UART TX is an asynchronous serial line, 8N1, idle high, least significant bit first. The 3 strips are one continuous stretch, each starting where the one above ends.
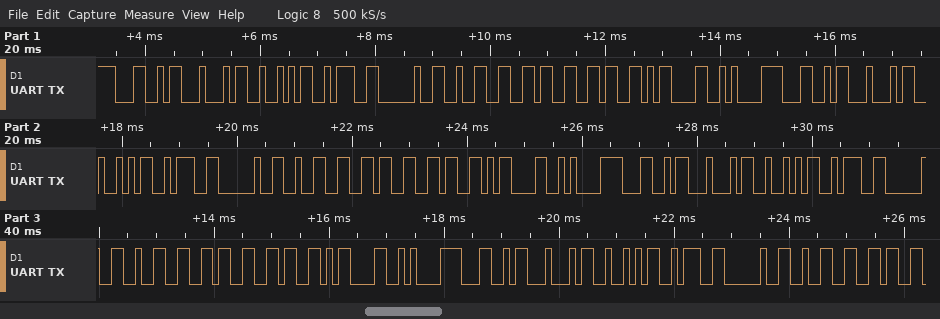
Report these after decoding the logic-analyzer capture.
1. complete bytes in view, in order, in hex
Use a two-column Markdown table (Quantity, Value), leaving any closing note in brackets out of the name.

| Quantity | Value |
|---|---|
| complete bytes in view, in order, in hex | 4C 44 52 3A 20 32 36 36 0D 0A 4C 44 52 3A 20 32 36 36 0D 0A 4C 44 52 3A 20 32 36 36 0D 0A 4C 44 52 3A 20 32 36 |
